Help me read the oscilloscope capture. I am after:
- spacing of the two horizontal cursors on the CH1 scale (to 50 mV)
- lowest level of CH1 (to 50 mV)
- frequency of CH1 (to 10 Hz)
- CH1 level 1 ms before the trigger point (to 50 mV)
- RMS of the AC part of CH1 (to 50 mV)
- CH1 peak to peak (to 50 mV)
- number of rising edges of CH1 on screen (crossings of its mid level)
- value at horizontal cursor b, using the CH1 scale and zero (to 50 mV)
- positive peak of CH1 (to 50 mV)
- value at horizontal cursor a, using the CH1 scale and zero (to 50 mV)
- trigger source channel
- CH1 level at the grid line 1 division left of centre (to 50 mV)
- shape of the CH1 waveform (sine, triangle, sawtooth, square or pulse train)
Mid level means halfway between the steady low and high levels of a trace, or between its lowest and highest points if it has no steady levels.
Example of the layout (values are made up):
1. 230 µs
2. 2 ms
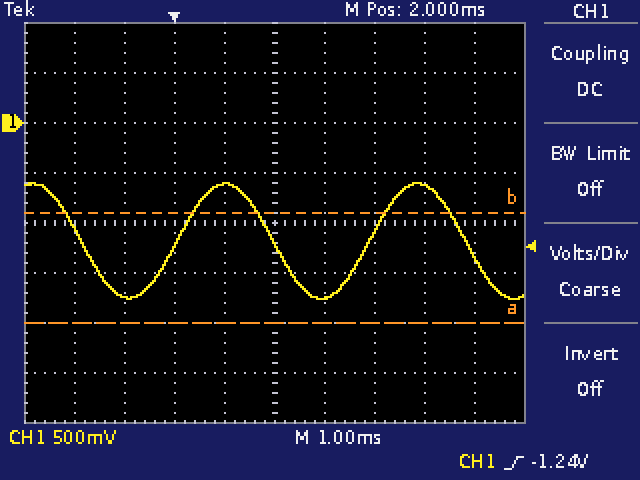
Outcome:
1. 1.10 V
2. -1.75 V
3. 260 Hz
4. -1.75 V
5. 400 mV
6. 1.15 V
7. 2
8. -900 mV
9. -600 mV
10. -2.00 V
11. CH1
12. -600 mV
13. sine
